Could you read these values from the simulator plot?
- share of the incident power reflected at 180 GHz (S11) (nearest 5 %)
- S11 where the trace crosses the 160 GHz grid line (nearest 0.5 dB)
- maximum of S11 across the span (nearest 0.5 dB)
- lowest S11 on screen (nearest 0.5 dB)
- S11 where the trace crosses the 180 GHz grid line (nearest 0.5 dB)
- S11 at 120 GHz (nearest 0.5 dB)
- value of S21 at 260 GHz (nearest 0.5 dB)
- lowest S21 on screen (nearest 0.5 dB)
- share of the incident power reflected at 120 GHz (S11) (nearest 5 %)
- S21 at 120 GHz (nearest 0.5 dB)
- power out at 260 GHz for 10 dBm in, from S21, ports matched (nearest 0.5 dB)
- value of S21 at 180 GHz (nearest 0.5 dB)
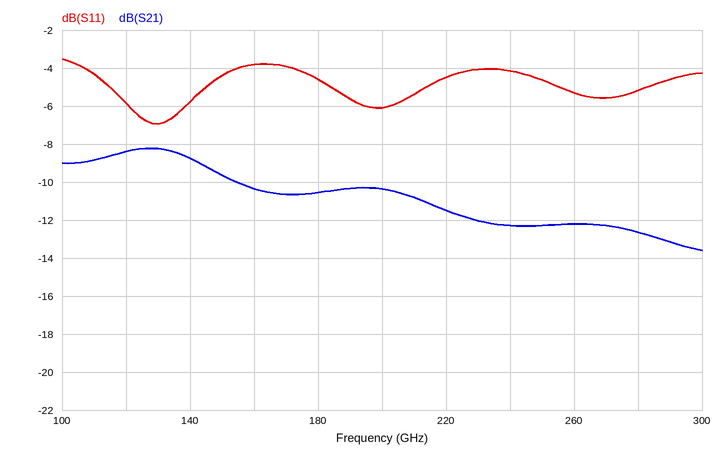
35 %
-4.0 dB
-3.5 dB
-7.0 dB
-4.5 dB
-6.0 dB
-12.0 dB
-13.5 dB
25 %
-8.5 dB
-2.0 dBm
-10.5 dB
